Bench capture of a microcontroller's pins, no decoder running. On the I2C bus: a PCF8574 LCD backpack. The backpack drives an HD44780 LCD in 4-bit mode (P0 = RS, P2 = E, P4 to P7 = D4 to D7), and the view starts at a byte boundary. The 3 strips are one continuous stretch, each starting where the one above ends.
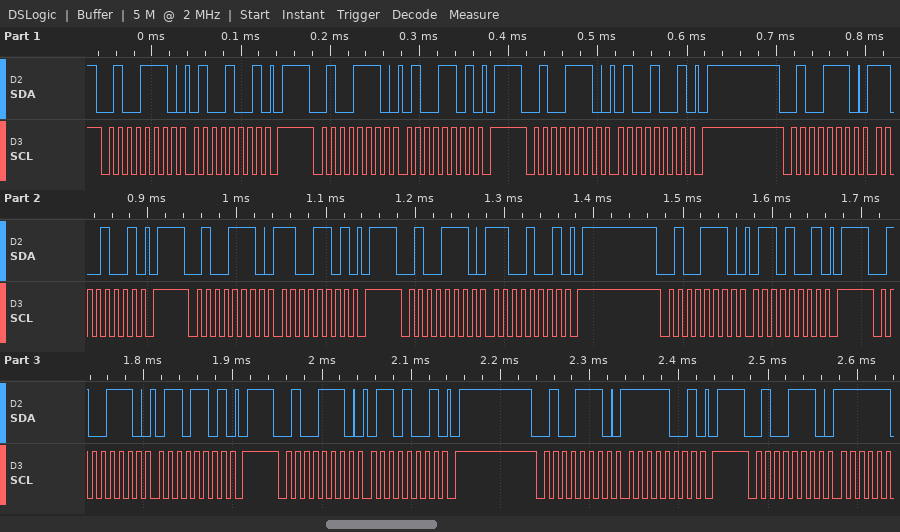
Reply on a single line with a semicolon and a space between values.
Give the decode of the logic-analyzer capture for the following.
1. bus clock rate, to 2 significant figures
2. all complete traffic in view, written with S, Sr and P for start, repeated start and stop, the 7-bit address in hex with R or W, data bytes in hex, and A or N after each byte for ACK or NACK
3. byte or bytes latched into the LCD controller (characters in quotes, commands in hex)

100 kHz; S 27W A 49 A P S 27W A 4D A P S 27W A 49 A P S 27W A C9 A P S 27W A CD A P S 27W A C9 A P S 27W A 69 A P S 27W A 6D A P S 27W A 69 A P S 27W A F9 A P S 27W A; 'L'
